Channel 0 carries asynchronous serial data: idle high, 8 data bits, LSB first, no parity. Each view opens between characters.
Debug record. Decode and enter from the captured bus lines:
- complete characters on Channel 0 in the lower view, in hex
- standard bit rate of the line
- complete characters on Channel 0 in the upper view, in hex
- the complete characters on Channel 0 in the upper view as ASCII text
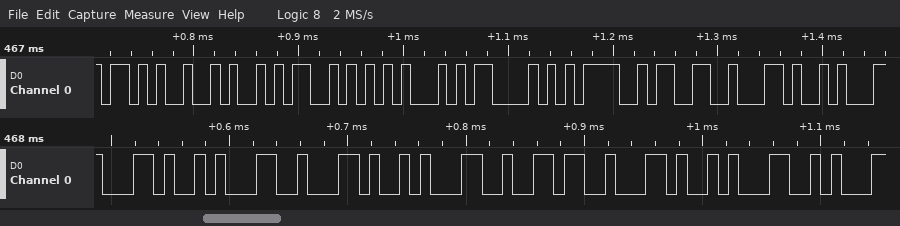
2C, 31, 2C, 31, 36, 2C, 31
115200 baud
2B, 4A, 53, 45, 43, 3D, 33, 2C
"+JSEC=3,"
